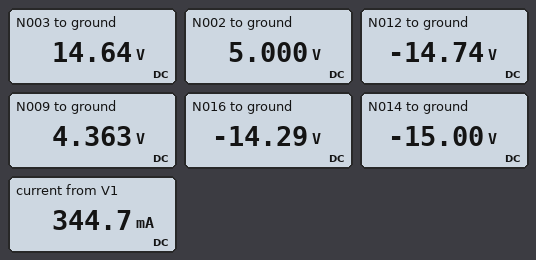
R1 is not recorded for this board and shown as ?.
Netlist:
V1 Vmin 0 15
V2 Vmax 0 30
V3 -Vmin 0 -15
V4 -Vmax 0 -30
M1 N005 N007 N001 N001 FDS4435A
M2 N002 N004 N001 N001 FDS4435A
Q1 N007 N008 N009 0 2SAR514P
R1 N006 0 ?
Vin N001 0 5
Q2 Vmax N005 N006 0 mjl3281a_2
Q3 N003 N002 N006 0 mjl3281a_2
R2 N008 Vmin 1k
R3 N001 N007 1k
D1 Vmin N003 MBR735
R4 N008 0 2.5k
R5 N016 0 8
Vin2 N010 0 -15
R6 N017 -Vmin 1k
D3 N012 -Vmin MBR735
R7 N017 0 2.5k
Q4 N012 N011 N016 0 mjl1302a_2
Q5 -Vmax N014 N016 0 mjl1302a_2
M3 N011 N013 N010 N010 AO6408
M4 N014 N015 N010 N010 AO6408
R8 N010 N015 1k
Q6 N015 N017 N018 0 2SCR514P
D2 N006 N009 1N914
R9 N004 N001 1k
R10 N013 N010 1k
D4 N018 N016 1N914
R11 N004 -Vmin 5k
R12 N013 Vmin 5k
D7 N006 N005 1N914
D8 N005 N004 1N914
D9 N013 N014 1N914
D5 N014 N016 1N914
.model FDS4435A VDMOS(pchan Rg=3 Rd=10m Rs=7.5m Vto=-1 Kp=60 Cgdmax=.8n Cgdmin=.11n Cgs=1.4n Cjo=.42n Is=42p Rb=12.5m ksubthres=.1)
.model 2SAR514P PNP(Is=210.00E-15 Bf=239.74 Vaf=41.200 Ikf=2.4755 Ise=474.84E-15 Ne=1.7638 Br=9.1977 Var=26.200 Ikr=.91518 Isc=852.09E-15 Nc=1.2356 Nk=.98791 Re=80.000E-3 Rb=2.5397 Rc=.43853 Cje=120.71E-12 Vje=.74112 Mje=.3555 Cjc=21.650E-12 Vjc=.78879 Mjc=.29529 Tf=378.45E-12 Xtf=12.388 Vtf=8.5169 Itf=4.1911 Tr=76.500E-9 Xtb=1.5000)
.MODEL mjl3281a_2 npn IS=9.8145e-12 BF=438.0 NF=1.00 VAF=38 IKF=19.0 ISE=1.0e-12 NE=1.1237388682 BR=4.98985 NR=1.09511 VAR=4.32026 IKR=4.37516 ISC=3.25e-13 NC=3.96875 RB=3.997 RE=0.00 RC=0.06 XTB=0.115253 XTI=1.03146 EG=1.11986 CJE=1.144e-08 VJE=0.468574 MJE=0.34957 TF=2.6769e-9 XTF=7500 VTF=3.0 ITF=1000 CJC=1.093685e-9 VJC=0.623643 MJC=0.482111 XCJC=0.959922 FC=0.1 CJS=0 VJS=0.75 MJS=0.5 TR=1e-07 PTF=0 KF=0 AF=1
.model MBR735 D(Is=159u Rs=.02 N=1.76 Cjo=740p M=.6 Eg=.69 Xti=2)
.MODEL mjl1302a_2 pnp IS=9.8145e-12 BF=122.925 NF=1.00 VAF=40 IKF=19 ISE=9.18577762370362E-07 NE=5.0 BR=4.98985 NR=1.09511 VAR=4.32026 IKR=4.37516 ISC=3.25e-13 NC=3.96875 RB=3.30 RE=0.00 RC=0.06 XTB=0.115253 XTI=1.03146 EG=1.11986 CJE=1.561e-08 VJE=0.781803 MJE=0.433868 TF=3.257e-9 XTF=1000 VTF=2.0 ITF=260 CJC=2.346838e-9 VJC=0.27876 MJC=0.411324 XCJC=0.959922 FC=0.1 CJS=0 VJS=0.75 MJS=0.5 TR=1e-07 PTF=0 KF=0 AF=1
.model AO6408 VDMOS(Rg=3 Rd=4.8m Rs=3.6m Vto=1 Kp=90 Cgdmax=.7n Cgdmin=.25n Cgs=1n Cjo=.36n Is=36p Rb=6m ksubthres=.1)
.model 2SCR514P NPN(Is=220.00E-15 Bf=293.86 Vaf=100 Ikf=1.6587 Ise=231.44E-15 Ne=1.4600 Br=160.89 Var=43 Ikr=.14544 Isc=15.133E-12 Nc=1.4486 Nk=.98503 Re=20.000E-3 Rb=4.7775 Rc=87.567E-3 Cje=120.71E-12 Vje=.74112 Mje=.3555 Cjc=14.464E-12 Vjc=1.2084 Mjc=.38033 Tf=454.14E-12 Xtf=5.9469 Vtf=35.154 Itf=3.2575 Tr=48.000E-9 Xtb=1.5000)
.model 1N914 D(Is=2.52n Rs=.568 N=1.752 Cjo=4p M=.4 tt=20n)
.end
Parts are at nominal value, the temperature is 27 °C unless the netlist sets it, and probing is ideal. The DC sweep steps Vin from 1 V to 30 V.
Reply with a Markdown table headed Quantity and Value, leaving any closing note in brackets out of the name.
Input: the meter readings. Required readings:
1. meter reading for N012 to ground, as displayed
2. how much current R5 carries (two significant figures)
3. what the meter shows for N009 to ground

| Quantity | Value |
|---|---|
| meter reading for N012 to ground, as displayed | -14.74 V |
| how much current R5 carries | 1.8 A |
| what the meter shows for N009 to ground | 4.363 V |
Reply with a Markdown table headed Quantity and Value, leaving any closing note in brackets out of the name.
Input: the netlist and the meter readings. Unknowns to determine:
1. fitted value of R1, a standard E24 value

| Quantity | Value |
|---|---|
| fitted value of R1, a standard E24 value | 13 Ω |
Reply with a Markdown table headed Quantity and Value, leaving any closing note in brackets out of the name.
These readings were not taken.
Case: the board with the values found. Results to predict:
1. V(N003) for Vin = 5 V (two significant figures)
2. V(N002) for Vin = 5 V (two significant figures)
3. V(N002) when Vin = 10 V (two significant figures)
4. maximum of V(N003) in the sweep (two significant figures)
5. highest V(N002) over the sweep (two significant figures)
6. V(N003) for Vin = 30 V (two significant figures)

| Quantity | Value |
|---|---|
| V(N003) for Vin = 5 V | 15 V |
| V(N002) for Vin = 5 V | 5.0 V |
| V(N002) when Vin = 10 V | 10 V |
| maximum of V(N003) in the sweep | 29 V |
| highest V(N002) over the sweep | 30 V |
| V(N003) for Vin = 30 V | 29 V |
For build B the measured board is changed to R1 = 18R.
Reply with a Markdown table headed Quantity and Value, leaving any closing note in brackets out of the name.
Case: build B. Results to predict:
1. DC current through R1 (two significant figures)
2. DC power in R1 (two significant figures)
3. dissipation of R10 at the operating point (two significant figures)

| Quantity | Value |
|---|---|
| DC current through R1 | 240 mA |
| DC power in R1 | 1.1 W |
| dissipation of R10 at the operating point | 440 µW |
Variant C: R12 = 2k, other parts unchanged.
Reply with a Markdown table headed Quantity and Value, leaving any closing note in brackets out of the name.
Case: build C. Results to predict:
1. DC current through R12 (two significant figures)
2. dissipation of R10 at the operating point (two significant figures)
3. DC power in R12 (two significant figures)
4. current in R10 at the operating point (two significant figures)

| Quantity | Value |
|---|---|
| DC current through R12 | 15 mA |
| dissipation of R10 at the operating point | 510 µW |
| DC power in R12 | 430 mW |
| current in R10 at the operating point | 710 µA |
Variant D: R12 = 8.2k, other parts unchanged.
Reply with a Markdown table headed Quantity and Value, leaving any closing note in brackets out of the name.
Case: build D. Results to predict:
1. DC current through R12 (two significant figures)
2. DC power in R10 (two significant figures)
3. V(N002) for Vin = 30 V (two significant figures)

| Quantity | Value |
|---|---|
| DC current through R12 | 3.6 mA |
| DC power in R10 | 400 µW |
| V(N002) for Vin = 30 V | 30 V |
